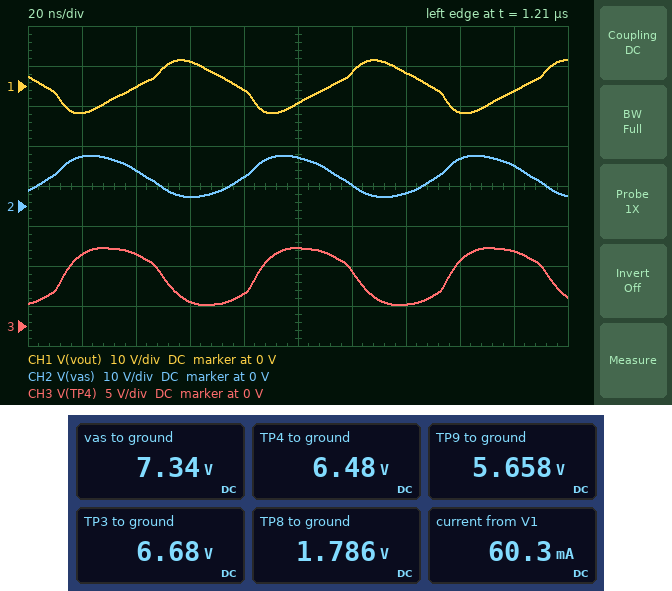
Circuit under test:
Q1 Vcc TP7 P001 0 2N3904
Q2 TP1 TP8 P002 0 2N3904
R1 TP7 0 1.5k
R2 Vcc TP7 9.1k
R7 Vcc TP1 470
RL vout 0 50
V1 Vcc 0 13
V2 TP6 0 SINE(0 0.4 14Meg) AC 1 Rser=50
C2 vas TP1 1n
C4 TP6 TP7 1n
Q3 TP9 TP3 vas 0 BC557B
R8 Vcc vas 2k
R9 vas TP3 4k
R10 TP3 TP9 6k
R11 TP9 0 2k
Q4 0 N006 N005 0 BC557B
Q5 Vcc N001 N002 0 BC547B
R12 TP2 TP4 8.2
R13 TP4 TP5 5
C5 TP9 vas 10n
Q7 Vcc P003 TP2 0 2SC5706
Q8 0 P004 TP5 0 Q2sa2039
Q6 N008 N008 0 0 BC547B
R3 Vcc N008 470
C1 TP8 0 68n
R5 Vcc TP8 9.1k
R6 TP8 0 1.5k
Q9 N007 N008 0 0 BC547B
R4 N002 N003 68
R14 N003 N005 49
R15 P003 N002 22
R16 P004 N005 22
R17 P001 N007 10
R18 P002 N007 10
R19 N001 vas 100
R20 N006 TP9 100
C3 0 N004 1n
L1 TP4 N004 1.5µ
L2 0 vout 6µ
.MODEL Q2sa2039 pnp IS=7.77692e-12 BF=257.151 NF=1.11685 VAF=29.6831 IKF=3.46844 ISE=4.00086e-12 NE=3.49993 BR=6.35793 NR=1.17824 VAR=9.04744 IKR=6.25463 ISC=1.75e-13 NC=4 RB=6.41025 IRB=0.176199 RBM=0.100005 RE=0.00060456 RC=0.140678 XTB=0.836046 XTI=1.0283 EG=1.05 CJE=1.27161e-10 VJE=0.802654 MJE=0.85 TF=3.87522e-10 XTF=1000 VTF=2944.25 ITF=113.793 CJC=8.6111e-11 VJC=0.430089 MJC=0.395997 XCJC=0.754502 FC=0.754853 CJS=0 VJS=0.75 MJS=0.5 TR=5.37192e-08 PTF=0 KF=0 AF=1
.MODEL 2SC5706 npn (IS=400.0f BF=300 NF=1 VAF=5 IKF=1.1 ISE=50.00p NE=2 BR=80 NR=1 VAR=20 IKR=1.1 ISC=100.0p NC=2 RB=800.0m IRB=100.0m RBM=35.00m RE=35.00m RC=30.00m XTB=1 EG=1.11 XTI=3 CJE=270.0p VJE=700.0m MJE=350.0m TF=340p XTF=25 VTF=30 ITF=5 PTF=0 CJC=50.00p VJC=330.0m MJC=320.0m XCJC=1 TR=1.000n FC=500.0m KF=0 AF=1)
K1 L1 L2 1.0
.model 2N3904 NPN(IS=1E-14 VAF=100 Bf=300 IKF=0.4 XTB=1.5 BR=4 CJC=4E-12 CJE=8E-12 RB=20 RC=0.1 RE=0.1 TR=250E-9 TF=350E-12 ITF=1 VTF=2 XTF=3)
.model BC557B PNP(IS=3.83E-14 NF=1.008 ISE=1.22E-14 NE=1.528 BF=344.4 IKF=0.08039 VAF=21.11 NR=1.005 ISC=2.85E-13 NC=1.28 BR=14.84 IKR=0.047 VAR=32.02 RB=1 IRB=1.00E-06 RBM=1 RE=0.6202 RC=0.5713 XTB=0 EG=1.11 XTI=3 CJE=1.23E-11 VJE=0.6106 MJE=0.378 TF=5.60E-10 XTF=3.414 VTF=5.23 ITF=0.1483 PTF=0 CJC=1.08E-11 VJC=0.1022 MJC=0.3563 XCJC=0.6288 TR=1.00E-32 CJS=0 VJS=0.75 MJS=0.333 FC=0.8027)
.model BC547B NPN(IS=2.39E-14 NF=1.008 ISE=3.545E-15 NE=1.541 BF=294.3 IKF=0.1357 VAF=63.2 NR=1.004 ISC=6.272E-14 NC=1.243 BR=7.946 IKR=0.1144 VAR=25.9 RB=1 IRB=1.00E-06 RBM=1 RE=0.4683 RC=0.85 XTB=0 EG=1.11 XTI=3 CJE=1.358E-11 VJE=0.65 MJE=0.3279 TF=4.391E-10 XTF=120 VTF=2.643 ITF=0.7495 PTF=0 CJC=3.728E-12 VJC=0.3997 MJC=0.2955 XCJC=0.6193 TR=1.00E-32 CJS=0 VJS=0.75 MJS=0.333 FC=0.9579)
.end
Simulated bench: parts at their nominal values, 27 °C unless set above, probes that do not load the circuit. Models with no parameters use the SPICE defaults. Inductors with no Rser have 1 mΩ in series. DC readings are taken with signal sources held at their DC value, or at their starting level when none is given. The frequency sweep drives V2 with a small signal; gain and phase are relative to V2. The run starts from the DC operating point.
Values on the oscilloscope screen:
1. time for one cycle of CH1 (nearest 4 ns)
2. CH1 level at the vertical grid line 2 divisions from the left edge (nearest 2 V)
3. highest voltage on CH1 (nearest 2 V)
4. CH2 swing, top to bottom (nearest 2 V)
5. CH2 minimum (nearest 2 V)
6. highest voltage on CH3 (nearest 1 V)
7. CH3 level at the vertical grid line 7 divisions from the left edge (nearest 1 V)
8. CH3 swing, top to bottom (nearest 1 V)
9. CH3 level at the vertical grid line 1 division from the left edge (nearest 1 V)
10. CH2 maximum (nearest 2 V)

72 ns
0 V
6 V
10 V
2 V
10 V
3 V
7 V
9 V
12 V
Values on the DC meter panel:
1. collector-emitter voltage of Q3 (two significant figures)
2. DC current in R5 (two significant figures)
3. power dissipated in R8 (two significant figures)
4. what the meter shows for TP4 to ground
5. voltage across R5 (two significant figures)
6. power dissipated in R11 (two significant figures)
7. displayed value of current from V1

-1.7 V
1.2 mA
16 mW
6.48 V
11 V
16 mW
60.3 mA
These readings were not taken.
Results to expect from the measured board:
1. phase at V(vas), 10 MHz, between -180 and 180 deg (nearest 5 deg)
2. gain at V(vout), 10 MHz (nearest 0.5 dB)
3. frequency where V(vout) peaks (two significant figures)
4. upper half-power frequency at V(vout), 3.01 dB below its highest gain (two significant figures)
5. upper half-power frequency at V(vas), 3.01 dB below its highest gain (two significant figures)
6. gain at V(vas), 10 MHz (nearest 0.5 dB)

-35 deg
15.5 dB
13 MHz
22 MHz
17 MHz
23.0 dB
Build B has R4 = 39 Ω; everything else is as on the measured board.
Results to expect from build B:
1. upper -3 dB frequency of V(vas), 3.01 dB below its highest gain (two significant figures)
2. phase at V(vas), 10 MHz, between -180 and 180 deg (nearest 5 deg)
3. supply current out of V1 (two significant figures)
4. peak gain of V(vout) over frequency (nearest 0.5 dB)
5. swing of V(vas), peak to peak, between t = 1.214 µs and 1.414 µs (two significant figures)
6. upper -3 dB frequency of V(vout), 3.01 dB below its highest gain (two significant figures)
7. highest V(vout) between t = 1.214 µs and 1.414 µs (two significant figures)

18 MHz
-30 deg
61 mA
16.5 dB
11 V
23 MHz
6.5 V
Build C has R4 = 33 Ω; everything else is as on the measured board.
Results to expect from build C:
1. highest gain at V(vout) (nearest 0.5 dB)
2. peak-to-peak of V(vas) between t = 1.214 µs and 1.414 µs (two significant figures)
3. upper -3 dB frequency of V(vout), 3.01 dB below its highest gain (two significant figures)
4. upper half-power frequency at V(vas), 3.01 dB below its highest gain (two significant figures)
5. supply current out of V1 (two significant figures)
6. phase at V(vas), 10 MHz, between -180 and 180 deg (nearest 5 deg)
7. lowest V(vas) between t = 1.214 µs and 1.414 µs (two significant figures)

16.5 dB
11 V
23 MHz
18 MHz
61 mA
-30 deg
2.1 V
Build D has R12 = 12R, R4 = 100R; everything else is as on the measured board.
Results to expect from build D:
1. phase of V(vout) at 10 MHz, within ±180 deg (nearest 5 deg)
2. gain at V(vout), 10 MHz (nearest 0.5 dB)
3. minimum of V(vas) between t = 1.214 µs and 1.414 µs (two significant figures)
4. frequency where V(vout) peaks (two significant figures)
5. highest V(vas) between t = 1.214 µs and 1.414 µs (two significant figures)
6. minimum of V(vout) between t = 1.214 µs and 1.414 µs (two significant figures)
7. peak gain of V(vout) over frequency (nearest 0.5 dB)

-160 deg
15.0 dB
2.3 V
12 MHz
12 V
-6.0 V
15.5 dB
